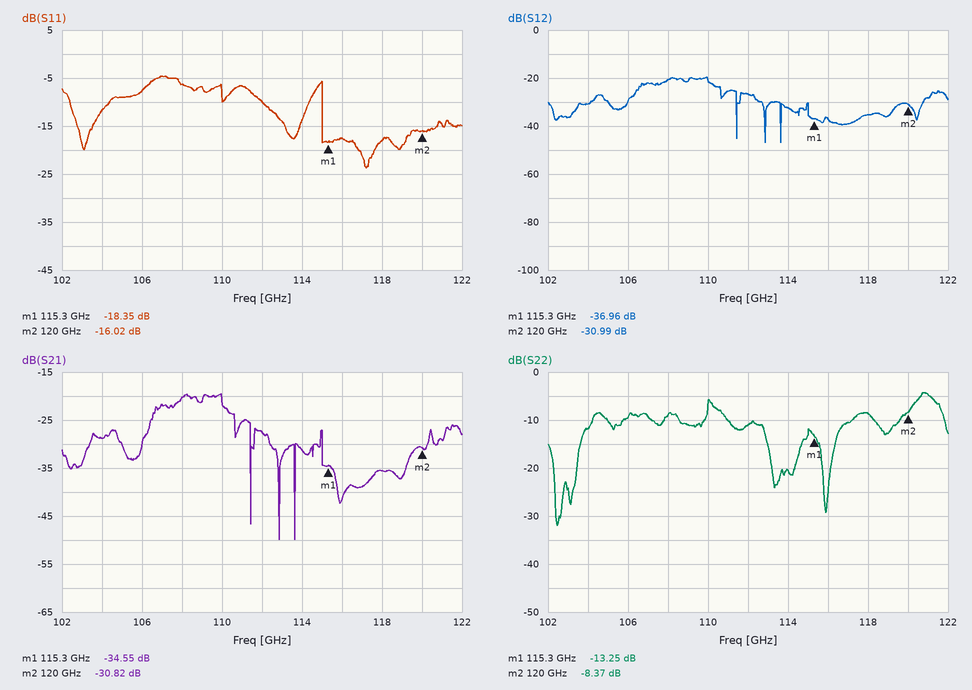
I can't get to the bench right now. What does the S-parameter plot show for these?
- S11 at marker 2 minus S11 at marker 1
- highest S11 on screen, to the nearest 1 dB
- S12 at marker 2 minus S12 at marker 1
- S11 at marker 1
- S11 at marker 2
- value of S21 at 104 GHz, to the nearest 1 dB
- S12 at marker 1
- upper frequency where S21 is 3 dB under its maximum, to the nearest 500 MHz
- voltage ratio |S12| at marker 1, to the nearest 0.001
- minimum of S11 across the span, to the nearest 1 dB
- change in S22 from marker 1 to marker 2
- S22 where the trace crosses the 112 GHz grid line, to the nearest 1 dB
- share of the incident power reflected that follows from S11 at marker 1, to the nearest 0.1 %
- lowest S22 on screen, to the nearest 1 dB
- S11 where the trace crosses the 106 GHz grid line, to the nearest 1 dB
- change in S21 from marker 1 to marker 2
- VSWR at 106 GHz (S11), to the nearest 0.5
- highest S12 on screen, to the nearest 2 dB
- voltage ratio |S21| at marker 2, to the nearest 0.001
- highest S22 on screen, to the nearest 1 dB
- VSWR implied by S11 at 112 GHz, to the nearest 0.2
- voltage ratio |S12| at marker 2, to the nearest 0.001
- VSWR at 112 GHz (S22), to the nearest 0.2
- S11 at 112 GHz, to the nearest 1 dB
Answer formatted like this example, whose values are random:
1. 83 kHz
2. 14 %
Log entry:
1. 2.33 dB
2. -5 dB
3. 5.97 dB
4. -18.35 dB
5. -16.02 dB
6. -29 dB
7. -36.96 dB
8. 110.0 GHz
9. 0.014
10. -24 dB
11. 4.88 dB
12. -11 dB
13. 1.5 %
14. -32 dB
15. -8 dB
16. 3.73 dB
17. 2.5
18. -20 dB
19. 0.029
20. -4 dB
21. 2.0
22. 0.028
23. 1.8
24. -10 dB
